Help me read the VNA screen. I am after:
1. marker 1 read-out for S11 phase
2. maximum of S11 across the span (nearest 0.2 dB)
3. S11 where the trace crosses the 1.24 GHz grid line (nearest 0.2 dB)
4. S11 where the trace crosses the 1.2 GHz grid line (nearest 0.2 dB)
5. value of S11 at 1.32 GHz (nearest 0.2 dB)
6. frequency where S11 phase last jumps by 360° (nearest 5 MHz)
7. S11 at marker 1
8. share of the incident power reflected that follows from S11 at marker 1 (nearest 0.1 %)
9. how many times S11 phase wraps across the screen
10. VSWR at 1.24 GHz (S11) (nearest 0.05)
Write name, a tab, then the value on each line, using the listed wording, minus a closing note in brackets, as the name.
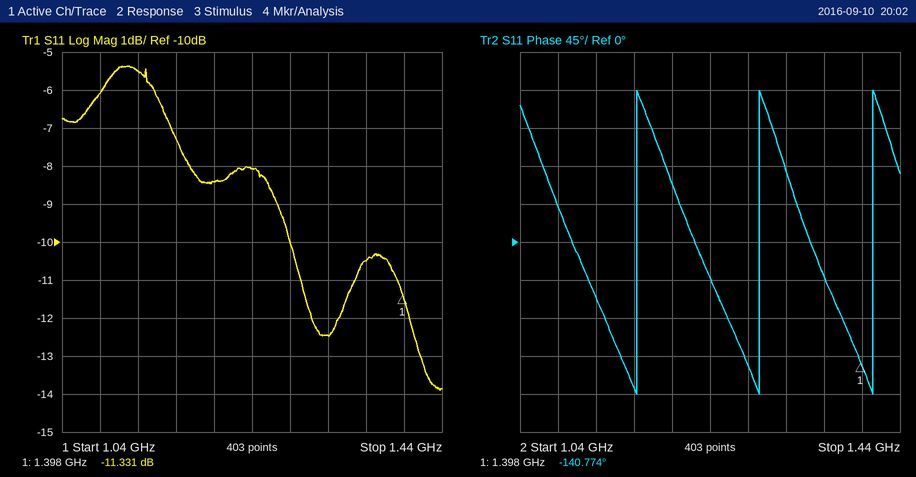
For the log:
marker 1 read-out for S11 phase	-140.774°
maximum of S11 across the span	-5.4 dB
S11 where the trace crosses the 1.24 GHz grid line	-8.0 dB
S11 where the trace crosses the 1.2 GHz grid line	-8.4 dB
value of S11 at 1.32 GHz	-12.4 dB
frequency where S11 phase last jumps by 360°	1.410 GHz
S11 at marker 1	-11.331 dB
share of the incident power reflected that follows from S11 at marker 1	7.4 %
how many times S11 phase wraps across the screen	3
VSWR at 1.24 GHz (S11)	2.30
